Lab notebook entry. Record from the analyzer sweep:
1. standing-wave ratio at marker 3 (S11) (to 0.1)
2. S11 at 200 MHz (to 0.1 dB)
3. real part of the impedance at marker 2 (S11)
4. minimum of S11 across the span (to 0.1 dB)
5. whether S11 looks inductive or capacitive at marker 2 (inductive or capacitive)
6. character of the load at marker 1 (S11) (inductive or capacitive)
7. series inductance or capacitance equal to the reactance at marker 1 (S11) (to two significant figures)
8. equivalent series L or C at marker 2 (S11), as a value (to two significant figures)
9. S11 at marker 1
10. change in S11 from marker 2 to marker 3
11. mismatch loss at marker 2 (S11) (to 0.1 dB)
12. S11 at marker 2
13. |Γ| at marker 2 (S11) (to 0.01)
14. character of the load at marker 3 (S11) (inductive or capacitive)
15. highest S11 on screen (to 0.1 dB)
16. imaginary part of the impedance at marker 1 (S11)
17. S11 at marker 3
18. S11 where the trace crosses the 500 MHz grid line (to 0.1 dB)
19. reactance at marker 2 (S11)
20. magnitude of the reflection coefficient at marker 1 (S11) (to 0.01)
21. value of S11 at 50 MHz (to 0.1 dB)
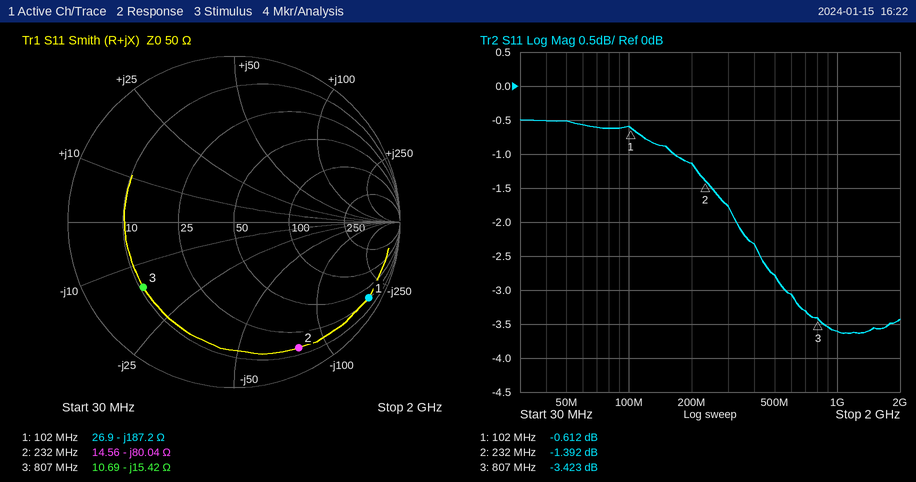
5.1
-1.1 dB
14.56 Ω
-3.6 dB
capacitive
capacitive
8.3 pF
8.6 pF
-0.612 dB
-2.031 dB
5.6 dB
-1.392 dB
0.85
capacitive
-0.5 dB
-187.2 Ω
-3.423 dB
-2.8 dB
-80.04 Ω
0.93
-0.5 dB
